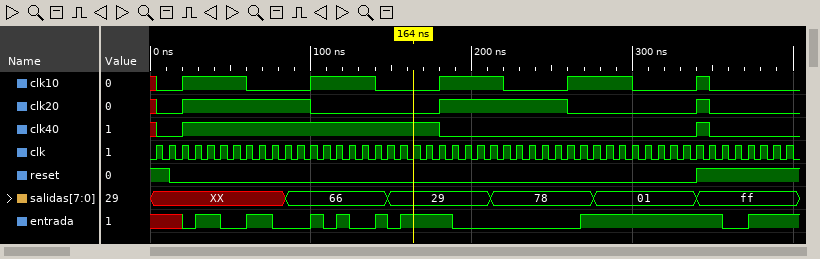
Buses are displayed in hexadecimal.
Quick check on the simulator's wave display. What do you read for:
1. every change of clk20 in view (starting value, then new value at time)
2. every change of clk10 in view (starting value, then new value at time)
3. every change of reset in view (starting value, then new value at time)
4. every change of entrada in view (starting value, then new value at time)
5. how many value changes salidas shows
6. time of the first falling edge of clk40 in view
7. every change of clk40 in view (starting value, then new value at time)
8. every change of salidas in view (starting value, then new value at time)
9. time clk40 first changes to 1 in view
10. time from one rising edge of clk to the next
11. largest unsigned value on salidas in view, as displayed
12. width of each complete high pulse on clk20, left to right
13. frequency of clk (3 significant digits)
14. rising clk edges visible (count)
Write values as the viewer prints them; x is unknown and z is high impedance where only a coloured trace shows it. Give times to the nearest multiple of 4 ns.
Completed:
x, 0 at 4 ns, 1 at 20 ns, 0 at 100 ns, 1 at 180 ns, 0 at 260 ns, 1 at 340 ns, 0 at 348 ns
x, 0 at 4 ns, 1 at 20 ns, 0 at 60 ns, 1 at 100 ns, 0 at 140 ns, 1 at 180 ns, 0 at 220 ns, 1 at 260 ns, 0 at 300 ns, 1 at 340 ns, 0 at 348 ns
1, 0 at 12 ns, 1 at 340 ns
x, 0 at 20 ns, 1 at 28 ns, 0 at 44 ns, 1 at 60 ns, 0 at 76 ns, 1 at 100 ns, 0 at 108 ns, 1 at 116 ns, 0 at 124 ns, 1 at 140 ns, 0 at 148 ns, 1 at 156 ns, 0 at 188 ns, 1 at 268 ns, 0 at 356 ns, 1 at 372 ns
5
180 ns
x, 0 at 4 ns, 1 at 20 ns, 0 at 180 ns, 1 at 340 ns, 0 at 348 ns
XX, 66 at 84 ns, 29 at 148 ns, 78 at 212 ns, 01 at 276 ns, ff at 340 ns
20 ns
8 ns
ff
80 ns, 80 ns, 8 ns
125 MHz
50
